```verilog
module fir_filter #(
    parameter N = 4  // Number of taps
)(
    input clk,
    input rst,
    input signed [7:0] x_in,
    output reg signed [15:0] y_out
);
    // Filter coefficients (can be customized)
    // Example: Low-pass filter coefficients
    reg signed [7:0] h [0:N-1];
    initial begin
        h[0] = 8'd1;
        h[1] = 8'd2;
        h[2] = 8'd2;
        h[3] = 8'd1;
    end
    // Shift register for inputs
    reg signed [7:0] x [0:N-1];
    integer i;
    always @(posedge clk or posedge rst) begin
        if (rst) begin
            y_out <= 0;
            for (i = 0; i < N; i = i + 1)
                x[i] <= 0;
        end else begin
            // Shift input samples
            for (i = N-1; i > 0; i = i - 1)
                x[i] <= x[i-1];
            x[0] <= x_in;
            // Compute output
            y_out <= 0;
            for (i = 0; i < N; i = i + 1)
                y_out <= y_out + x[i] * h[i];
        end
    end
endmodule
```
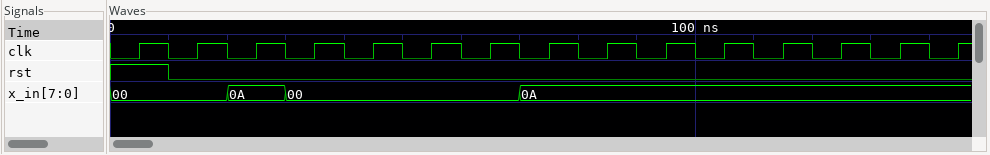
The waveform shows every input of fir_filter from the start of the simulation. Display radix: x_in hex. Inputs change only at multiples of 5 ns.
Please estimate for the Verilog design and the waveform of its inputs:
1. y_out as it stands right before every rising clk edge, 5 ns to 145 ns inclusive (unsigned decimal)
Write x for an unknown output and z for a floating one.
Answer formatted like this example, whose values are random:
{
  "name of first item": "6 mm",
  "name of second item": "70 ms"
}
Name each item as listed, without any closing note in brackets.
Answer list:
{
  "y_out as it stands right before every rising clk edge, 5 ns to 145 ns inclusive": "0, 0, 0, 0, 0, 0, 0, 10, 10, 10, 10, 10, 20, 30, 40"
}
